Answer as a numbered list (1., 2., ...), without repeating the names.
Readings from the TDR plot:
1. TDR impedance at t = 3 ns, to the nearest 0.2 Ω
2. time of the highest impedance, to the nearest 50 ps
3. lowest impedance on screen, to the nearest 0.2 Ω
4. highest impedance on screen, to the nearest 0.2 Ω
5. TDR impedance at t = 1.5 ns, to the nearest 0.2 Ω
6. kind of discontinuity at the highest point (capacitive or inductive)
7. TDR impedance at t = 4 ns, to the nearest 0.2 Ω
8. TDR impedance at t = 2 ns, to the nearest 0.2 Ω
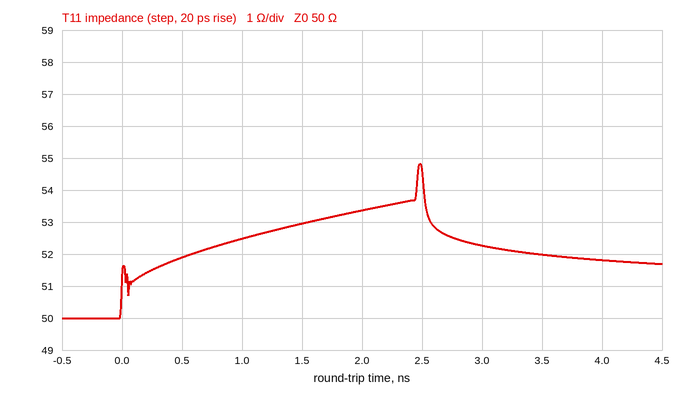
1. 52.2 Ω
2. 2.50 ns
3. 50.0 Ω
4. 54.8 Ω
5. 53.0 Ω
6. inductive
7. 51.8 Ω
8. 53.4 Ω
